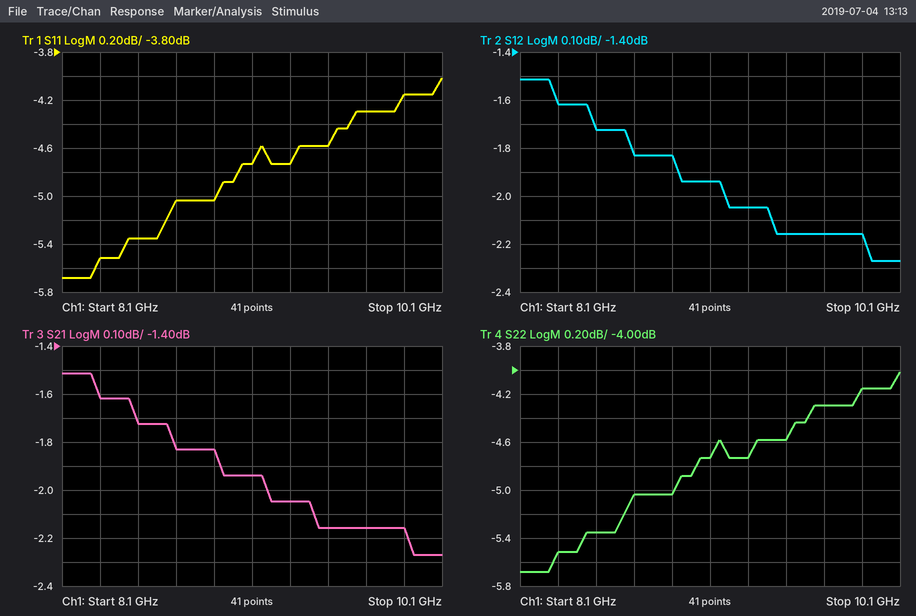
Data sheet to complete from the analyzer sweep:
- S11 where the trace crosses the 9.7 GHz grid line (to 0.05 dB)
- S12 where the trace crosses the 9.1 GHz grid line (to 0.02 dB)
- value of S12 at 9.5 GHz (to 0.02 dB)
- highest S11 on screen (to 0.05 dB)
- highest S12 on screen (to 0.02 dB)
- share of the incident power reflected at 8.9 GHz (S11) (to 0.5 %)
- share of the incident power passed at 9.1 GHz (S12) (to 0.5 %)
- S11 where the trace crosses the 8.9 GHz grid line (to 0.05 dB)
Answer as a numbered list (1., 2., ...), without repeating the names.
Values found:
1. -4.30 dB
2. -1.94 dB
3. -2.16 dB
4. -4.00 dB
5. -1.52 dB
6. 31.5 %
7. 64.0 %
8. -5.05 dB
